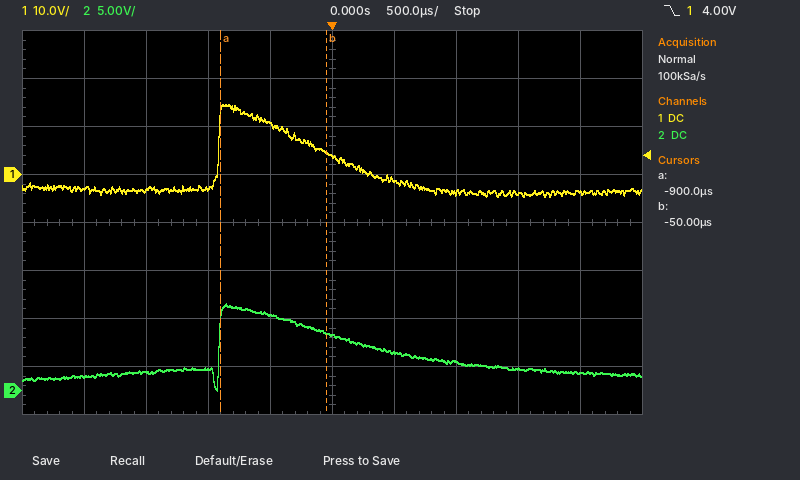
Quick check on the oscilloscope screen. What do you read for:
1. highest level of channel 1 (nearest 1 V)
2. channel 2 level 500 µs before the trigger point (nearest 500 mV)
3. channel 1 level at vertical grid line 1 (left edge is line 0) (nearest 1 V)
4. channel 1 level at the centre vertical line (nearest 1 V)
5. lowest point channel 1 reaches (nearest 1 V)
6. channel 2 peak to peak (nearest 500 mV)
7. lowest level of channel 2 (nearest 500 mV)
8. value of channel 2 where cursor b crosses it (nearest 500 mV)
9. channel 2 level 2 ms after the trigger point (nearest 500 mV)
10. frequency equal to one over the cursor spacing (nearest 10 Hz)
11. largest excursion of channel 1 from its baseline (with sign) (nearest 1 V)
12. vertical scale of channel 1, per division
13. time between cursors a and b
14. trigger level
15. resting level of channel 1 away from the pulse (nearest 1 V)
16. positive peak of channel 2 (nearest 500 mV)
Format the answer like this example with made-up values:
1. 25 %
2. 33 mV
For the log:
1. 15 V
2. 8.0 V
3. -3 V
4. 4 V
5. -5 V
6. 9.0 V
7. 0.0 V
8. 6.0 V
9. 2.0 V
10. 1.18 kHz
11. +18 V
12. 10 V
13. 850 µs
14. 4.00 V
15. -3 V
16. 9.0 V
